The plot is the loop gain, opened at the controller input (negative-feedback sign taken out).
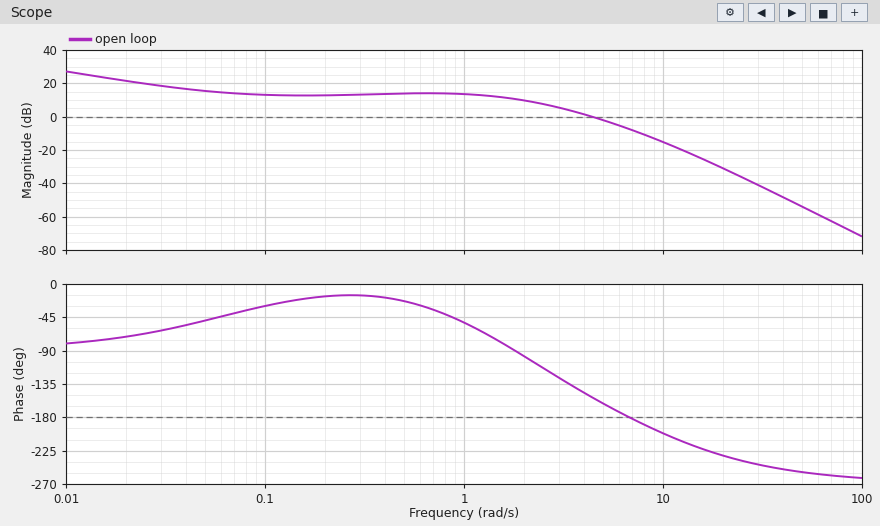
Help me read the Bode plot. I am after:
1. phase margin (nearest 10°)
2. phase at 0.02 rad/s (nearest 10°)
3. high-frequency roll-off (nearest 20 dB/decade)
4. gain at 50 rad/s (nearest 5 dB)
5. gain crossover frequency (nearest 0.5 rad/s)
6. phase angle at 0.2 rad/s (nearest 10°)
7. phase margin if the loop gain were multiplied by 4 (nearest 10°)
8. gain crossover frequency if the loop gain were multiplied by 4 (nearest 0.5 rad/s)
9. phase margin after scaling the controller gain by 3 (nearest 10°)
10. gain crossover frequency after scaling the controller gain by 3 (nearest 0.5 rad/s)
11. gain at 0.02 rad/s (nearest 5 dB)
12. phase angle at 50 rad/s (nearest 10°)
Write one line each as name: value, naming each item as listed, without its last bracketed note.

phase margin: 30°
phase at 0.02 rad/s: -70°
high-frequency roll-off: -60 dB/decade
gain at 50 rad/s: -55 dB
gain crossover frequency: 4.5 rad/s
phase angle at 0.2 rad/s: -20°
phase margin if the loop gain were multiplied by 4: -10°
gain crossover frequency if the loop gain were multiplied by 4: 8.5 rad/s
phase margin after scaling the controller gain by 3: -10°
gain crossover frequency after scaling the controller gain by 3: 7.5 rad/s
gain at 0.02 rad/s: 20 dB
phase angle at 50 rad/s: -250°
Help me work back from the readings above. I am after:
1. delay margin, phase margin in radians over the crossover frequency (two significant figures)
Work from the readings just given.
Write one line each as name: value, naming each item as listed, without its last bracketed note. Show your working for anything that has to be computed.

delay margin, phase margin in radians over the crossover frequency: 30 × π / 180 / 4.5 = 0.12 s
